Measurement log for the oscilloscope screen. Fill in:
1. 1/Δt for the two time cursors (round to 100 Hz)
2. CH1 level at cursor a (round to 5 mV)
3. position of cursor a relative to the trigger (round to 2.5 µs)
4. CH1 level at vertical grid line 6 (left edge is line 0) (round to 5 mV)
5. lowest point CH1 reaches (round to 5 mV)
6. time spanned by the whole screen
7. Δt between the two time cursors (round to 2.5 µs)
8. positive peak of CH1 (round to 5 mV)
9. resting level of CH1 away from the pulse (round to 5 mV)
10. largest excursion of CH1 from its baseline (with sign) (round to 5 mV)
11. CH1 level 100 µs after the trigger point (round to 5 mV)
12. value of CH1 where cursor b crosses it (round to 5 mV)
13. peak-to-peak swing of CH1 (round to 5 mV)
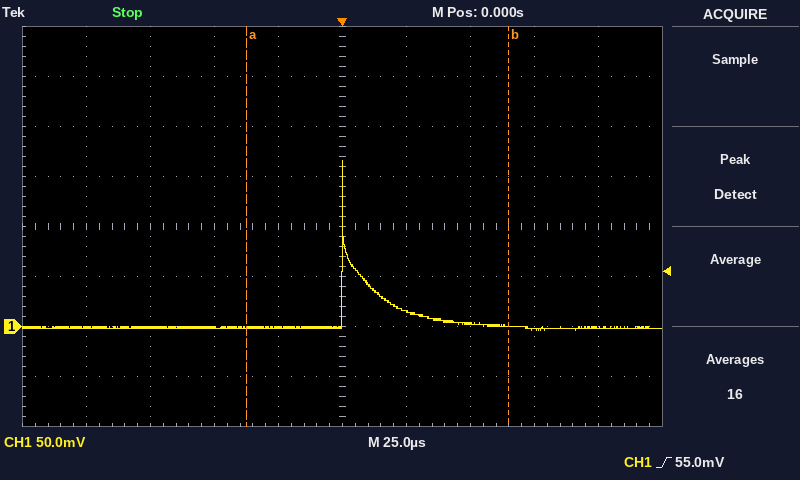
9.8 kHz
0 mV
-37.5 µs
15 mV
-5 mV
250 µs
102.5 µs
165 mV
0 mV
+165 mV
0 mV
0 mV
170 mV
